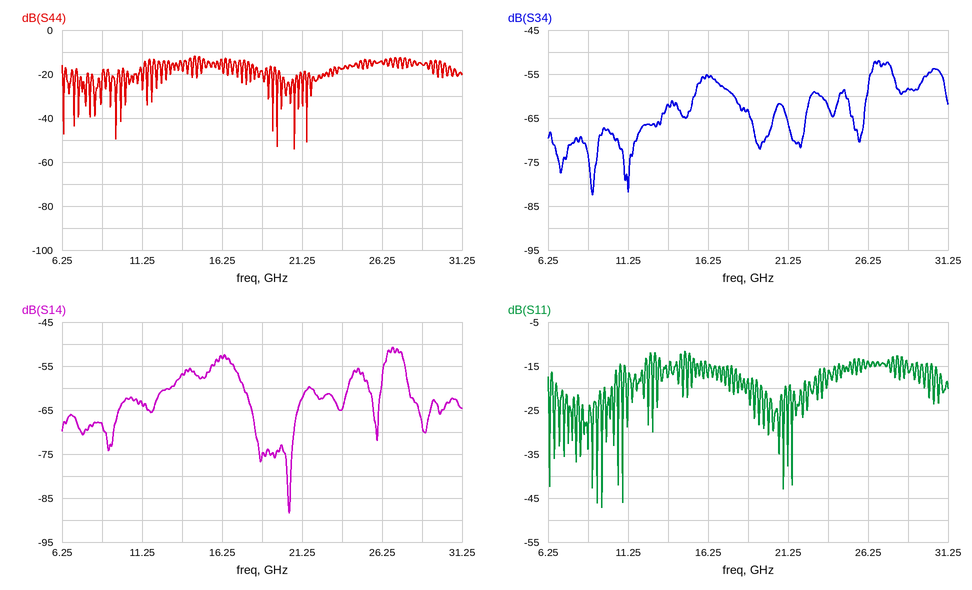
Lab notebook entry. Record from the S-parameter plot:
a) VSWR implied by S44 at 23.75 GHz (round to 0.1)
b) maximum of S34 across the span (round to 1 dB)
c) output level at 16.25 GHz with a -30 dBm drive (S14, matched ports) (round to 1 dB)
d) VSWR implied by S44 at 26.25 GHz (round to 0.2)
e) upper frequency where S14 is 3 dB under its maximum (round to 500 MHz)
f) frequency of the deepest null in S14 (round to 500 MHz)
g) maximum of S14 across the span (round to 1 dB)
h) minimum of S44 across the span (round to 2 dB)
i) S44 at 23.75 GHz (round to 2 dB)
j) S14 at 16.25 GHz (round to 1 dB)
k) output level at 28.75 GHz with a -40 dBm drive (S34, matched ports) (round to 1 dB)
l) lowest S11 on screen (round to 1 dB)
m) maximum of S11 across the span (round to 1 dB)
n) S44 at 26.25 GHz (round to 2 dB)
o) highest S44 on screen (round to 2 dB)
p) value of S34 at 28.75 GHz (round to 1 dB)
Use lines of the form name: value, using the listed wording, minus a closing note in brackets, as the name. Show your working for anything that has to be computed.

VSWR implied by S44 at 23.75 GHz: |Γ| = 10^(-18/20) = 0.1259; VSWR = (1 + 0.1259)/(1 − 0.1259) ≈ 1.3
maximum of S34 across the span: -52 dB
output level at 16.25 GHz with a -30 dBm drive (S14, matched ports): -30 dBm + (-53 dB) = -83 dBm
VSWR implied by S44 at 26.25 GHz: |Γ| = 10^(-14/20) = 0.1995; VSWR = (1 + 0.1995)/(1 − 0.1995) ≈ 1.50, so 1.4 to the nearest 0.2
upper frequency where S14 is 3 dB under its maximum: 27.5 GHz
frequency of the deepest null in S14: 20.5 GHz
maximum of S14 across the span: -51 dB
minimum of S44 across the span: -54 dB
S44 at 23.75 GHz: -18 dB
S14 at 16.25 GHz: -53 dB
output level at 28.75 GHz with a -40 dBm drive (S34, matched ports): -40 dBm + (-58 dB) = -98 dBm
lowest S11 on screen: -47 dB
maximum of S11 across the span: -12 dB
S44 at 26.25 GHz: -14 dB
highest S44 on screen: -12 dB
value of S34 at 28.75 GHz: -58 dB
